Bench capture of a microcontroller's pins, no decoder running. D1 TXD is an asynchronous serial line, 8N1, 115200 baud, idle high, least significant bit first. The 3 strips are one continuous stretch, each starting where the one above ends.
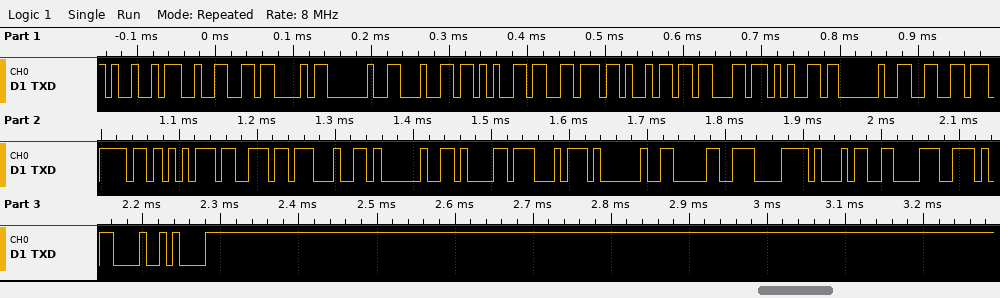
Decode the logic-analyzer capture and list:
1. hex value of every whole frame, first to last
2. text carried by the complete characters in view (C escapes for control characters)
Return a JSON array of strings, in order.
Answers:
["49 32 43 20 64 65 76 69 63 65 20 66 6F 75 6E 64 20 61 74 20 30 78 34 38 0D 0A", "\"I2C device found at 0x48\\r\\n\""]
